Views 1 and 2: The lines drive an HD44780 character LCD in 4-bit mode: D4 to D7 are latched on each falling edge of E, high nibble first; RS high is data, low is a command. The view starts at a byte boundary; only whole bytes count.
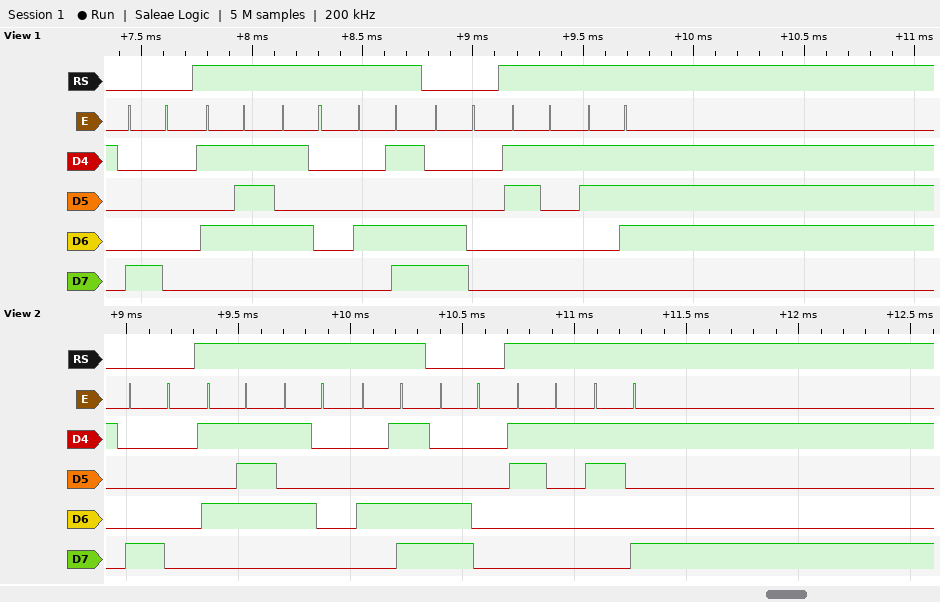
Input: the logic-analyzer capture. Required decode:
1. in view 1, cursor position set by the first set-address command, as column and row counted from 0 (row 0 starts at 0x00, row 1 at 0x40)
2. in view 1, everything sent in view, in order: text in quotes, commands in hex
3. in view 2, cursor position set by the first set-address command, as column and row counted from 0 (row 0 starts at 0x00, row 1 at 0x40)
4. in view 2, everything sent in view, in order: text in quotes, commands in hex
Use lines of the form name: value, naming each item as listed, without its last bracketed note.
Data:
in view 1, cursor position set by the first set-address command, as column and row counted from 0: column 0, row 0
in view 1, everything sent in view, in order: text in quotes, commands in hex: 0x80 "WPM" 0xC0 "17"
in view 2, cursor position set by the first set-address command, as column and row counted from 0: column 0, row 0
in view 2, everything sent in view, in order: text in quotes, commands in hex: 0x80 "WPM" 0xC0 "19"
